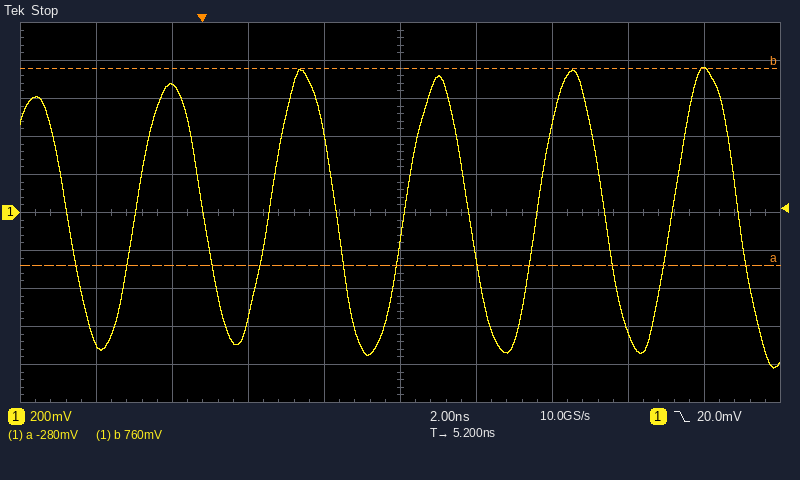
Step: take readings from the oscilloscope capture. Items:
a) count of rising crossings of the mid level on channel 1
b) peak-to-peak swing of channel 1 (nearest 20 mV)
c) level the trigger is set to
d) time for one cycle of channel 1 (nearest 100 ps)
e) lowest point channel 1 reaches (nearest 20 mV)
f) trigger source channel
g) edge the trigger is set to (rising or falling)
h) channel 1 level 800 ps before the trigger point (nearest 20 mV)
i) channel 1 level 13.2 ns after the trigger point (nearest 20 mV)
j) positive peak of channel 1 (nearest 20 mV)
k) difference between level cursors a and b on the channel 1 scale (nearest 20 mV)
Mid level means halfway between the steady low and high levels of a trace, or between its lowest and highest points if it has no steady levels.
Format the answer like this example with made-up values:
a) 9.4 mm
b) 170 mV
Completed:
a) 5
b) 1.58 V
c) 20.0 mV
d) 3.5 ns
e) -820 mV
f) channel 1
g) falling
h) 660 mV
i) 760 mV
j) 760 mV
k) 1.04 V
